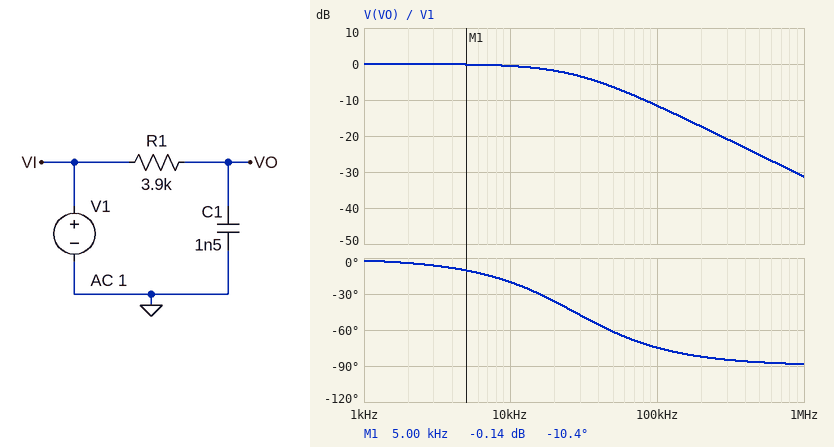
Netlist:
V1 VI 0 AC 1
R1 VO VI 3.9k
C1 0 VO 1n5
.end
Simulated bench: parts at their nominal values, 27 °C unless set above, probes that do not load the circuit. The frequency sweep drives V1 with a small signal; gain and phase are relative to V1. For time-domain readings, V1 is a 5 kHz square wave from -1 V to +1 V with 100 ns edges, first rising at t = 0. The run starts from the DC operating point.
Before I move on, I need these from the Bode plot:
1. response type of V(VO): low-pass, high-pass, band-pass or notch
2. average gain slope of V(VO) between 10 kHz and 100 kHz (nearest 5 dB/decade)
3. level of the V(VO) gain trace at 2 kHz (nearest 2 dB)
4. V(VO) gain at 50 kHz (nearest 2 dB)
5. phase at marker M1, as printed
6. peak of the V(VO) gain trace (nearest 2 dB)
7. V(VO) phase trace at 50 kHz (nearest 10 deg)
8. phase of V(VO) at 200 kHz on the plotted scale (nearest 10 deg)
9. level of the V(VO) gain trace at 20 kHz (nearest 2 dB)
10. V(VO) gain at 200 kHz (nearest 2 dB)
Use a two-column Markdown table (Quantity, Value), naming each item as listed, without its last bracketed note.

| Quantity | Value |
|---|---|
| response type of V(VO): low-pass, high-pass, band-pass or notch | low-pass |
| average gain slope of V(VO) between 10 kHz and 100 kHz | -10 dB/decade |
| level of the V(VO) gain trace at 2 kHz | 0 dB |
| V(VO) gain at 50 kHz | -6 dB |
| phase at marker M1, as printed | -10.4 deg |
| peak of the V(VO) gain trace | 0 dB |
| V(VO) phase trace at 50 kHz | -60 deg |
| phase of V(VO) at 200 kHz on the plotted scale | -80 deg |
| level of the V(VO) gain trace at 20 kHz | -2 dB |
| V(VO) gain at 200 kHz | -18 dB |
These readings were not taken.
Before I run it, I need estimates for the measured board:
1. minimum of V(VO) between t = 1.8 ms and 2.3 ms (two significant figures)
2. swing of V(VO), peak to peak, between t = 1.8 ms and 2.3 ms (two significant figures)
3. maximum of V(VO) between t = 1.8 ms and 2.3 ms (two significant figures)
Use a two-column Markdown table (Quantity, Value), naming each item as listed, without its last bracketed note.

| Quantity | Value |
|---|---|
| minimum of V(VO) between t = 1.8 ms and 2.3 ms | -1.0 V |
| swing of V(VO), peak to peak, between t = 1.8 ms and 2.3 ms | 2.0 V |
| maximum of V(VO) between t = 1.8 ms and 2.3 ms | 1.0 V |
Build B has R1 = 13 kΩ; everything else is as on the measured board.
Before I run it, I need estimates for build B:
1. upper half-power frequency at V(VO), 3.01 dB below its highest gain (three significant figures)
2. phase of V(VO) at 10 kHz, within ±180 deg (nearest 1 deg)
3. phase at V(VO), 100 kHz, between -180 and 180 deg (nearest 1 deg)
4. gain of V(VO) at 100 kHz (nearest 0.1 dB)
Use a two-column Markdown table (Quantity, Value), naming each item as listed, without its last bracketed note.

| Quantity | Value |
|---|---|
| upper half-power frequency at V(VO), 3.01 dB below its highest gain | 8.16 kHz |
| phase of V(VO) at 10 kHz, within ±180 deg | -51 deg |
| phase at V(VO), 100 kHz, between -180 and 180 deg | -85 deg |
| gain of V(VO) at 100 kHz | -21.8 dB |
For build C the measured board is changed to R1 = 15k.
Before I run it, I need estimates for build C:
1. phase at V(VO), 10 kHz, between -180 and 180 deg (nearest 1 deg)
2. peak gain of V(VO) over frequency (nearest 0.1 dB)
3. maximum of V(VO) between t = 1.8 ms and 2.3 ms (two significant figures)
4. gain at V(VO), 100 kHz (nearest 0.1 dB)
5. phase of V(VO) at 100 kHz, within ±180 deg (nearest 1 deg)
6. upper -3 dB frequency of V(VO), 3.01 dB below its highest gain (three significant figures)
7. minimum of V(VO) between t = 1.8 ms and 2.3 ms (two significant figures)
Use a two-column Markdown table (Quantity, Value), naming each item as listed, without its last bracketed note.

| Quantity | Value |
|---|---|
| phase at V(VO), 10 kHz, between -180 and 180 deg | -55 deg |
| peak gain of V(VO) over frequency | 0 dB |
| maximum of V(VO) between t = 1.8 ms and 2.3 ms | 980 mV |
| gain at V(VO), 100 kHz | -23.0 dB |
| phase of V(VO) at 100 kHz, within ±180 deg | -86 deg |
| upper -3 dB frequency of V(VO), 3.01 dB below its highest gain | 7.07 kHz |
| minimum of V(VO) between t = 1.8 ms and 2.3 ms | -980 mV |
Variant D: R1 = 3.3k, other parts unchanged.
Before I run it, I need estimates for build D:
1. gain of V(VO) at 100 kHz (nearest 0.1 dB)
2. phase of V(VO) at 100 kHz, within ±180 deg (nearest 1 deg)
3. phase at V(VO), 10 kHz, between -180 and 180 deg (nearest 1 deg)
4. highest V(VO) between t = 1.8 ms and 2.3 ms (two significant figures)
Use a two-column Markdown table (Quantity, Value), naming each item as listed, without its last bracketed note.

| Quantity | Value |
|---|---|
| gain of V(VO) at 100 kHz | -10.3 dB |
| phase of V(VO) at 100 kHz, within ±180 deg | -72 deg |
| phase at V(VO), 10 kHz, between -180 and 180 deg | -17 deg |
| highest V(VO) between t = 1.8 ms and 2.3 ms | 1.0 V |
